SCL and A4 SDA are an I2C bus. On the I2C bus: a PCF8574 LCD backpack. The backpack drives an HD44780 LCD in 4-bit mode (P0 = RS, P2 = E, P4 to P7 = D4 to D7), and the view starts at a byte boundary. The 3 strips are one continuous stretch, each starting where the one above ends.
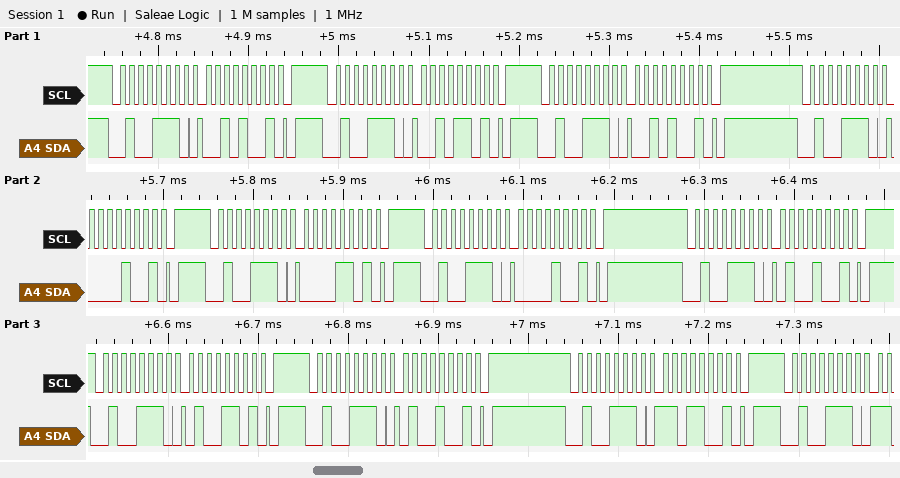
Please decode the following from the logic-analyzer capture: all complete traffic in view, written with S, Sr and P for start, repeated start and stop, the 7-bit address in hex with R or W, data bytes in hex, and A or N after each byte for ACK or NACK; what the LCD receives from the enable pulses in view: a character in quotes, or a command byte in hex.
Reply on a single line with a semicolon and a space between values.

S 27W A 29 A P S 27W A 2D A P S 27W A 29 A P S 27W A 09 A P S 27W A 0D A P S 27W A 09 A P S 27W A 49 A P S 27W A 4D A P S 27W A 49 A P S 27W A D9 A P S 27W A; ' '
